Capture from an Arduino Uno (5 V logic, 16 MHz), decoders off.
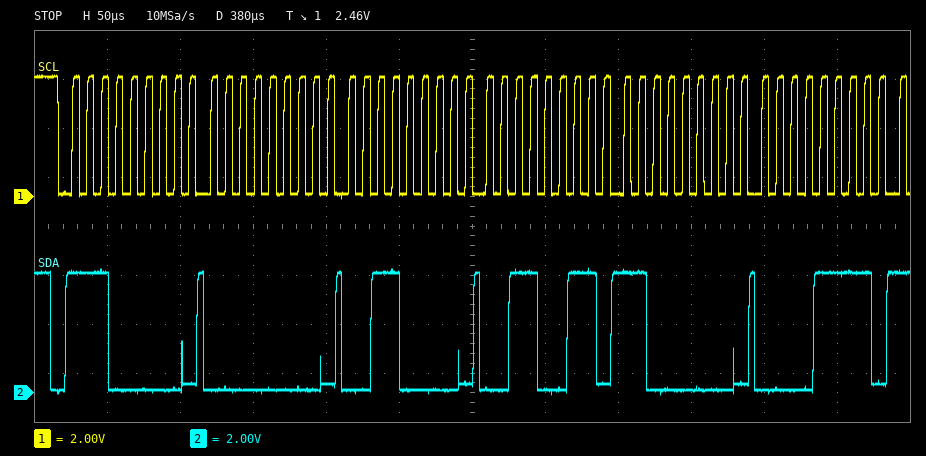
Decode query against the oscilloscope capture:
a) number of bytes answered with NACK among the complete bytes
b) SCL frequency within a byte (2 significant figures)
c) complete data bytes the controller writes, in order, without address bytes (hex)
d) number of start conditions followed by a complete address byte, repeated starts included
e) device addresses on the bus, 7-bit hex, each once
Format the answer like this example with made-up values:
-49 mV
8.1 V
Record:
0
100 kHz
00 30 33 C0 0F
1
0x70
